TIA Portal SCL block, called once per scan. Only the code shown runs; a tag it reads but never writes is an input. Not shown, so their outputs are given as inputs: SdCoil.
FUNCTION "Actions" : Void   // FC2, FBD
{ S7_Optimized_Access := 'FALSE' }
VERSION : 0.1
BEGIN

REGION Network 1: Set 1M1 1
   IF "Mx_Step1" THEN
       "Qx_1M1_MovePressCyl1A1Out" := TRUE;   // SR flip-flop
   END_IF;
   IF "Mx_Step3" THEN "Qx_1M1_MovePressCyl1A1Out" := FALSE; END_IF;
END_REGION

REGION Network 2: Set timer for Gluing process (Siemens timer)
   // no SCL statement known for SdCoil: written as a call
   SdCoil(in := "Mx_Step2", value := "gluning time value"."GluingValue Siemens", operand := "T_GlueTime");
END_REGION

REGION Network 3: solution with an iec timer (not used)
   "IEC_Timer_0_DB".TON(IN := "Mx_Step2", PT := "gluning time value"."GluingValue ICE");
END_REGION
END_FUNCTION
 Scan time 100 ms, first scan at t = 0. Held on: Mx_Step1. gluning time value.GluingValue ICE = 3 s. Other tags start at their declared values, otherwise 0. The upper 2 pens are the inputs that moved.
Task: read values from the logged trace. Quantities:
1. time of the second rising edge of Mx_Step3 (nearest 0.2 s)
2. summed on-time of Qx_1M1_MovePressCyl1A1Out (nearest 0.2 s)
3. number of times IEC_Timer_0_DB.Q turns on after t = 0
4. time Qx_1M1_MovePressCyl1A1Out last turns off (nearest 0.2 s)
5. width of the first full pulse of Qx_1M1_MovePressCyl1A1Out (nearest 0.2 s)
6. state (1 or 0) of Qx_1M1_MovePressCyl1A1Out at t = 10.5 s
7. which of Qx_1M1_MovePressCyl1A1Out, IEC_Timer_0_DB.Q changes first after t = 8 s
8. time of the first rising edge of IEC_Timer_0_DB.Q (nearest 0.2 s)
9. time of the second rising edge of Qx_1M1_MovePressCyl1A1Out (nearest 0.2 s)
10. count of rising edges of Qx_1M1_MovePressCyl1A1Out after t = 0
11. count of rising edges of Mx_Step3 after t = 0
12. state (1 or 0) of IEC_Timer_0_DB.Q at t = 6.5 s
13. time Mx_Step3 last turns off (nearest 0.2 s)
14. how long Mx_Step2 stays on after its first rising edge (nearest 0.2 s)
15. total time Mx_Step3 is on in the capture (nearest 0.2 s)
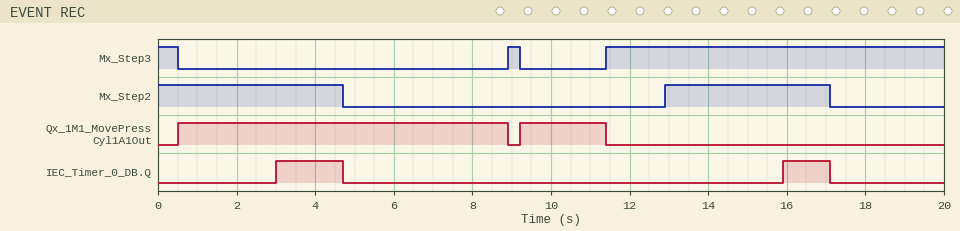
11.4 s
10.6 s
2
11.4 s
8.4 s
1
Qx_1M1_MovePressCyl1A1Out
3.0 s
9.2 s
2
2
0
9.2 s
4.2 s
9.4 s
